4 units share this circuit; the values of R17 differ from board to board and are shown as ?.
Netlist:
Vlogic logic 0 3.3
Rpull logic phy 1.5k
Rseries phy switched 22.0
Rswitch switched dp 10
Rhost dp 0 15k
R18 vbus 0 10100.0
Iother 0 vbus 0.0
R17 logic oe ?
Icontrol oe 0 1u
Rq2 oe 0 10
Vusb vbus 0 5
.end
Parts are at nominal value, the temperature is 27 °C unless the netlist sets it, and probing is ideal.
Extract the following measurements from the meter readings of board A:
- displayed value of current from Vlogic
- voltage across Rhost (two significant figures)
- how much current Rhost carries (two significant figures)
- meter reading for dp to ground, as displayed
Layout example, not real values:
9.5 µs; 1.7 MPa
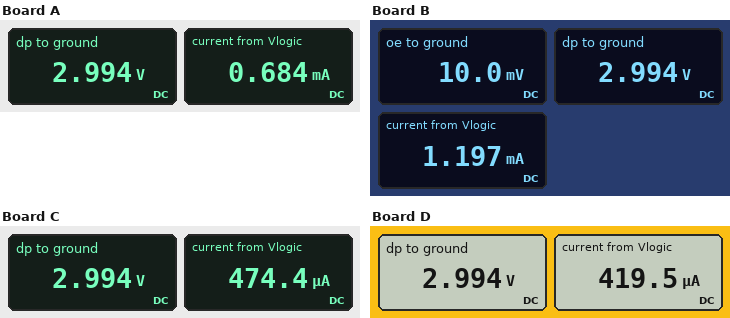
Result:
0.684 mA; 3.0 V; 200 µA; 2.994 V
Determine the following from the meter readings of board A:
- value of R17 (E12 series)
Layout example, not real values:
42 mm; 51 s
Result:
6.8 kΩ
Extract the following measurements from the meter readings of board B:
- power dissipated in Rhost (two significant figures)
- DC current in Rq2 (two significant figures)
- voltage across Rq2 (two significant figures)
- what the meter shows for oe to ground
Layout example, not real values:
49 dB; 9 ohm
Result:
600 µW; 1.0 mA; 10 mV; 10.0 mV
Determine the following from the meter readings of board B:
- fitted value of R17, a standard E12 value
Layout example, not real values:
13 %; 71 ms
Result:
3.3 kΩ
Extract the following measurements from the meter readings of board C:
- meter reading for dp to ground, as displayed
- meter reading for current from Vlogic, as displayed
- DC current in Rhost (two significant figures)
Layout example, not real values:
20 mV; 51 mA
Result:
2.994 V; 474.4 µA; 200 µA
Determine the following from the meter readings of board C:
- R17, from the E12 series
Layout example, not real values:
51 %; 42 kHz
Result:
12 kΩ
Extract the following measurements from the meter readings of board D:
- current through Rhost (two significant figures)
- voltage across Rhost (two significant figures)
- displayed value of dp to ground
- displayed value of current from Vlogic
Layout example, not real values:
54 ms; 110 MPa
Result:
200 µA; 3.0 V; 2.994 V; 419.5 µA
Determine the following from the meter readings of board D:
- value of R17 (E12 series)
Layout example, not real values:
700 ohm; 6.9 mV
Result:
15 kΩ
